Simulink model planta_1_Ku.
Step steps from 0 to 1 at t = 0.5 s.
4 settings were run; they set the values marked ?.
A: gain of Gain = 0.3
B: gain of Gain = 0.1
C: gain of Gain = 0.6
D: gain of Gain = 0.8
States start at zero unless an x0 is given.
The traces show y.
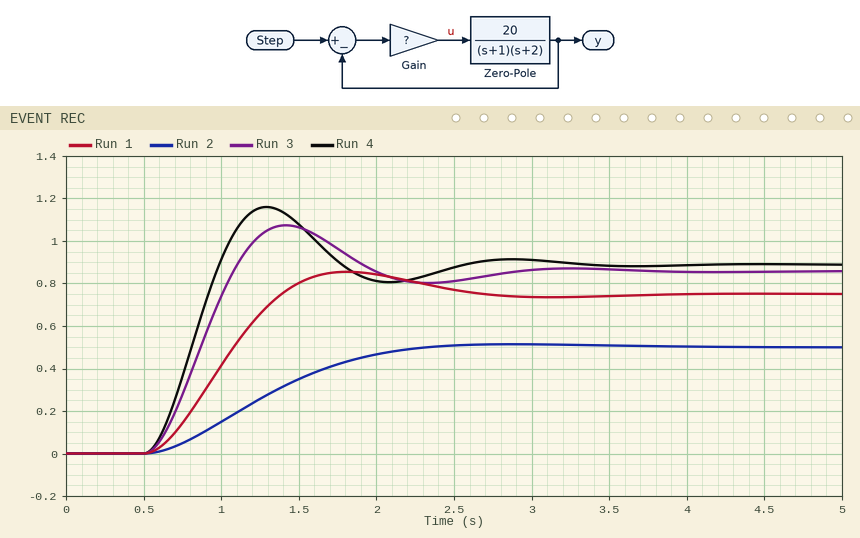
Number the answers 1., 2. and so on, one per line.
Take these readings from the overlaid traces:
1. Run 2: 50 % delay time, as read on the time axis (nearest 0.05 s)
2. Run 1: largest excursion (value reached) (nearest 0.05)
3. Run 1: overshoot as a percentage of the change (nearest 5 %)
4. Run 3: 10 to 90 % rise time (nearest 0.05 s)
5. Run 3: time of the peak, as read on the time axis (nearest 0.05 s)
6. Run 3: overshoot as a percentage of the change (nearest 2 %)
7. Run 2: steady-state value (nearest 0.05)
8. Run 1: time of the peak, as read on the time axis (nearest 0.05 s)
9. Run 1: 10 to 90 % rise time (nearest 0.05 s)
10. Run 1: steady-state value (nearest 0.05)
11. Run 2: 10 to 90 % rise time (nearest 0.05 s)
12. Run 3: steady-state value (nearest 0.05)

1. 1.25 s
2. 0.85
3. 15 %
4. 0.40 s
5. 1.40 s
6. 26 %
7. 0.50
8. 1.80 s
9. 0.60 s
10. 0.75
11. 1.15 s
12. 0.85
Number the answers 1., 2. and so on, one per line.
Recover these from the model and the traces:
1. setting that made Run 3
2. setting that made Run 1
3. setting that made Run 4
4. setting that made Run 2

1. C
2. A
3. D
4. B
